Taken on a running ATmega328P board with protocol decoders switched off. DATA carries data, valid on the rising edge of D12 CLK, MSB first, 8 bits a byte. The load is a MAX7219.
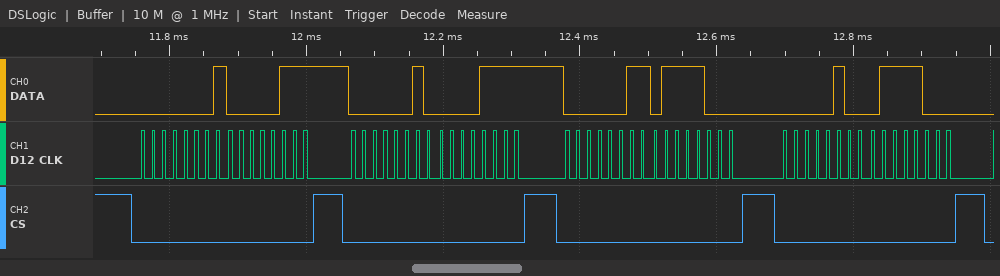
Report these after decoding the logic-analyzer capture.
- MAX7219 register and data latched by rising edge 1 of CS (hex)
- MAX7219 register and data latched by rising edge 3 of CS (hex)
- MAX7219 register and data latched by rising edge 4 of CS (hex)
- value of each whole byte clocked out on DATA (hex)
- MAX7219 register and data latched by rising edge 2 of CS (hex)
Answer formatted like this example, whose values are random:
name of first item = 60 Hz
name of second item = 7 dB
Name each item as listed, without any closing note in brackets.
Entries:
MAX7219 register and data latched by rising edge 1 of CS = register 0x1, data 0x07
MAX7219 register and data latched by rising edge 3 of CS = register 0x3, data 0x78
MAX7219 register and data latched by rising edge 4 of CS = register 0x4, data 0x78
value of each whole byte clocked out on DATA = 01 07 02 0F 03 78 04 78
MAX7219 register and data latched by rising edge 2 of CS = register 0x2, data 0x0F
